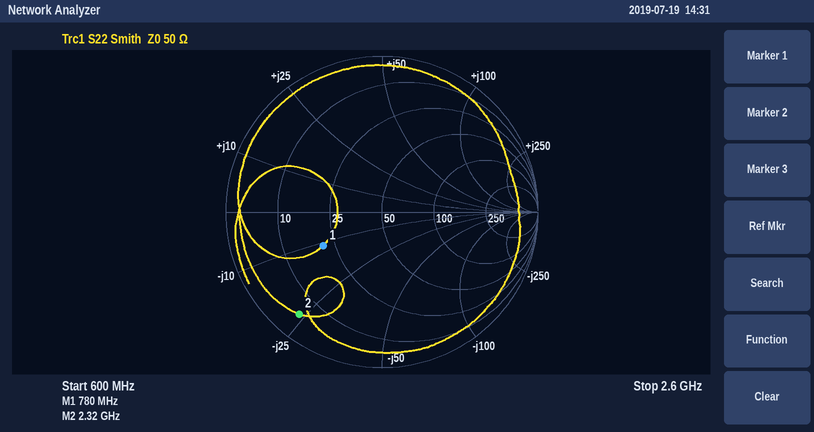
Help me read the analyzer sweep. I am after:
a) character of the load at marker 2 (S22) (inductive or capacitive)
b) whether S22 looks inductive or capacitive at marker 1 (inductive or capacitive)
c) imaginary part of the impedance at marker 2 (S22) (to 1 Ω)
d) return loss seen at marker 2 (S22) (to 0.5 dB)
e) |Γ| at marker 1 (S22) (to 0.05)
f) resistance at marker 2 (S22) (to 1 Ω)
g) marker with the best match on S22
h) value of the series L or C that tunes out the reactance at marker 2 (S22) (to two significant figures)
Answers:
capacitive
capacitive
-24 Ω
1.5 dB
0.45
5 Ω
marker 1
1.6 nH
